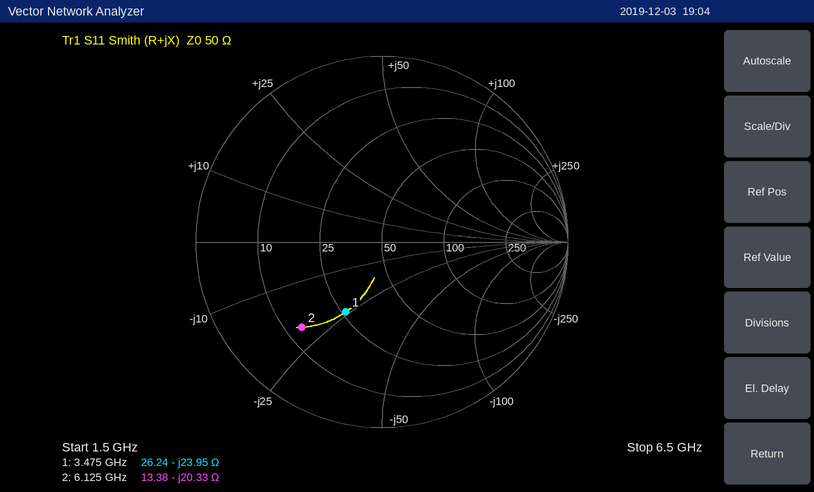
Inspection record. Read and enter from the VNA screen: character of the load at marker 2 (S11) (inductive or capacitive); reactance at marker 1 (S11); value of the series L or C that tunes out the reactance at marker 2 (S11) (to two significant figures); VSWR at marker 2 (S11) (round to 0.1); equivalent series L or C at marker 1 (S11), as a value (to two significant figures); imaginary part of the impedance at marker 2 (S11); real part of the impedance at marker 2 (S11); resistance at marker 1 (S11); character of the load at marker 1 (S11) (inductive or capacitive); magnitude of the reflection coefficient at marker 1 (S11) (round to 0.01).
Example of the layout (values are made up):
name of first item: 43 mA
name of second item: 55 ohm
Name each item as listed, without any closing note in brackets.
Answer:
character of the load at marker 2 (S11): capacitive
reactance at marker 1: -23.95 Ω
value of the series L or C that tunes out the reactance at marker 2 (S11): 530 pH
VSWR at marker 2 (S11): 4.4
equivalent series L or C at marker 1 (S11), as a value: 1.9 pF
imaginary part of the impedance at marker 2: -20.33 Ω
real part of the impedance at marker 2: 13.38 Ω
resistance at marker 1: 26.24 Ω
character of the load at marker 1 (S11): capacitive
magnitude of the reflection coefficient at marker 1 (S11): 0.42
